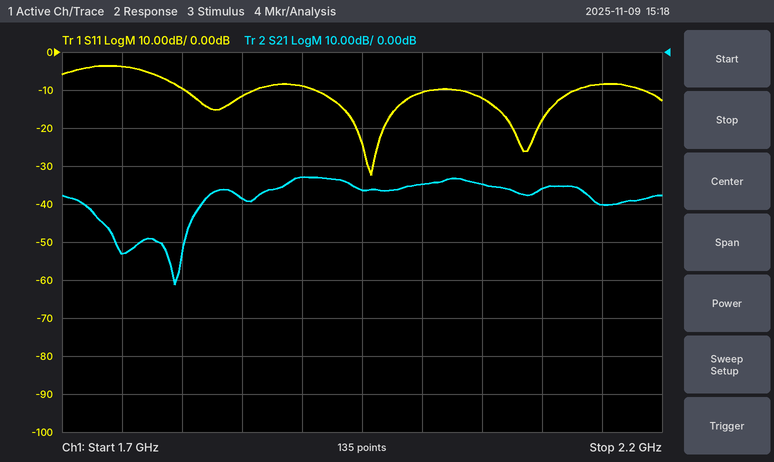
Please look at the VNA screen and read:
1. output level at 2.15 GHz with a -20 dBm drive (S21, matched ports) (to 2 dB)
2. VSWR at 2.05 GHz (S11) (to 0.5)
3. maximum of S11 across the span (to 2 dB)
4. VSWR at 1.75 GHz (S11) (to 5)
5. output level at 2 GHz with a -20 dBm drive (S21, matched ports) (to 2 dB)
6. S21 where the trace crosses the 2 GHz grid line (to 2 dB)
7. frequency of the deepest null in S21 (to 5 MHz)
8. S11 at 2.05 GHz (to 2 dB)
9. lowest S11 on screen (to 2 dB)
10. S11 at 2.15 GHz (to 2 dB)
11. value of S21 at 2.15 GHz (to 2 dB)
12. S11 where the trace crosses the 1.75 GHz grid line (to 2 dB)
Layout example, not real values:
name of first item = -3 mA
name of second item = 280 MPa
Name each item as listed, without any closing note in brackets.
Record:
output level at 2.15 GHz with a -20 dBm drive (S21, matched ports) = -60 dBm
VSWR at 2.05 GHz (S11) = 1.5
maximum of S11 across the span = -4 dB
VSWR at 1.75 GHz (S11) = 5
output level at 2 GHz with a -20 dBm drive (S21, matched ports) = -54 dBm
S21 where the trace crosses the 2 GHz grid line = -34 dB
frequency of the deepest null in S21 = 1.795 GHz
S11 at 2.05 GHz = -12 dB
lowest S11 on screen = -32 dB
S11 at 2.15 GHz = -8 dB
value of S21 at 2.15 GHz = -40 dB
S11 where the trace crosses the 1.75 GHz grid line = -4 dB
